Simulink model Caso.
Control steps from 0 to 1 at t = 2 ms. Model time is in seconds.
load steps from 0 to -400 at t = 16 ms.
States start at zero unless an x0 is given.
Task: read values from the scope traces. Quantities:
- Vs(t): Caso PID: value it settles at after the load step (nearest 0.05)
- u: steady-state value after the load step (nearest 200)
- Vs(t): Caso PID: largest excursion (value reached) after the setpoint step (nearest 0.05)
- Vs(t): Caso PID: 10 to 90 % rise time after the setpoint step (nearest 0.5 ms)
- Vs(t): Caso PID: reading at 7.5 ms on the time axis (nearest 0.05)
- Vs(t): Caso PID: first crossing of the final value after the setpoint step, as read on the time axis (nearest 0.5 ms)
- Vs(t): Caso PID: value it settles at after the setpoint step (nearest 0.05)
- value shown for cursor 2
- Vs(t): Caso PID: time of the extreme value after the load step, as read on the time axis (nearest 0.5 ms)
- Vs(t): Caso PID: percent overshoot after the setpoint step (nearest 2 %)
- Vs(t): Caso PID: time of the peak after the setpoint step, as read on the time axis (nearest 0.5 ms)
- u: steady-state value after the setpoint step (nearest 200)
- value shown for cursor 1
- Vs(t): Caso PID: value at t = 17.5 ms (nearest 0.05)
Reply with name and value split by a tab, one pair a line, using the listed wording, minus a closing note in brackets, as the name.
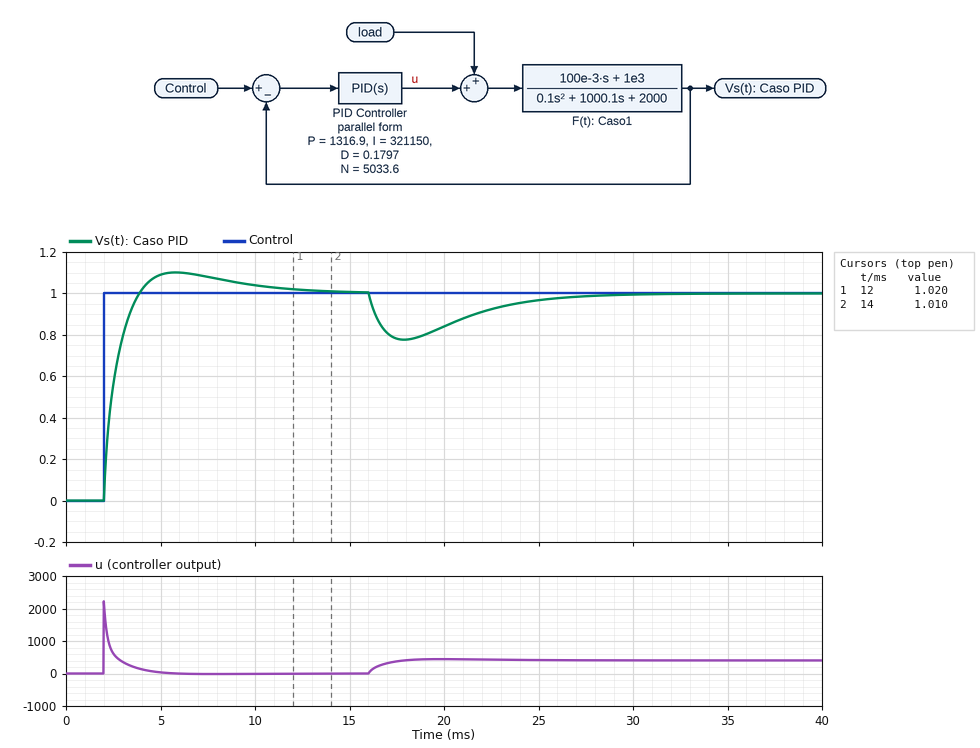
Vs(t): Caso PID: value it settles at after the load step	1.00
u: steady-state value after the load step	400
Vs(t): Caso PID: largest excursion (value reached) after the setpoint step	1.10
Vs(t): Caso PID: 10 to 90 % rise time after the setpoint step	1.5 ms
Vs(t): Caso PID: reading at 7.5 ms on the time axis	1.10
Vs(t): Caso PID: first crossing of the final value after the setpoint step, as read on the time axis	4.0 ms
Vs(t): Caso PID: value it settles at after the setpoint step	1.00
value shown for cursor 2	1.010
Vs(t): Caso PID: time of the extreme value after the load step, as read on the time axis	18.0 ms
Vs(t): Caso PID: percent overshoot after the setpoint step	10 %
Vs(t): Caso PID: time of the peak after the setpoint step, as read on the time axis	6.0 ms
u: steady-state value after the setpoint step	0
value shown for cursor 1	1.020
Vs(t): Caso PID: value at t = 17.5 ms	0.80
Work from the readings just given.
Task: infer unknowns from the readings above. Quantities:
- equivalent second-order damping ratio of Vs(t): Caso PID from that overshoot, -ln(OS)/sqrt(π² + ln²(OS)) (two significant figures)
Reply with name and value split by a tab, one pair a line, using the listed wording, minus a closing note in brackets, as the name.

equivalent second-order damping ratio of Vs(t): Caso PID from that overshoot, -ln(OS)/sqrt(π² + ln²(OS))	0.59
